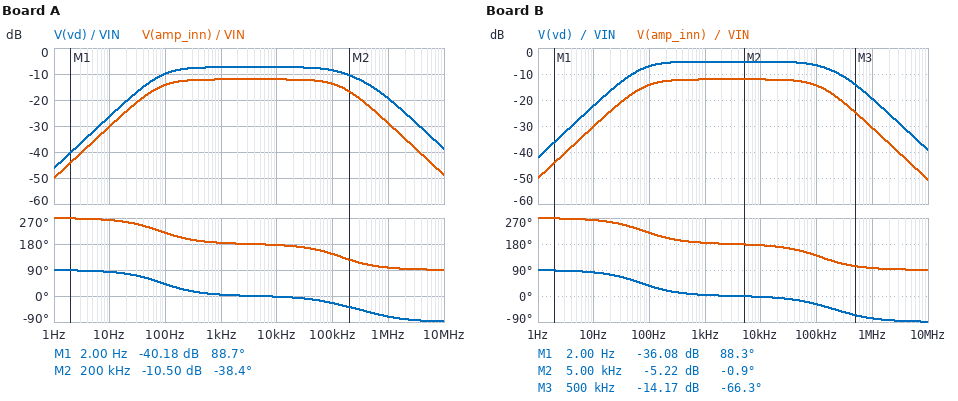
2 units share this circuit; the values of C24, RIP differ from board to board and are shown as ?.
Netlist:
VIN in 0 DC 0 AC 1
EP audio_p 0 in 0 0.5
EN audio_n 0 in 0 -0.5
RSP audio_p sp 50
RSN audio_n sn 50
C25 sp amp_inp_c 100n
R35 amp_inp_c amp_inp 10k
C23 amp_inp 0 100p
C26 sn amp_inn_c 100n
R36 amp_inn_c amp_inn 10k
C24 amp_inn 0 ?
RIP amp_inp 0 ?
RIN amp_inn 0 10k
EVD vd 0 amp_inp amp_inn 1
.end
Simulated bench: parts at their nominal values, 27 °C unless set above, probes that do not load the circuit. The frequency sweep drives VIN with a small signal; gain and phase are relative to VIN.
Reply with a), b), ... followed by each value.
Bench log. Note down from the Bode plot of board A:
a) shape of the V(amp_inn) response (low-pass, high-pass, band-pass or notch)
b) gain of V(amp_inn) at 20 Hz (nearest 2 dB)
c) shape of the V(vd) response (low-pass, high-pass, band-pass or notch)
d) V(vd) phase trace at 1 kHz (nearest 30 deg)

a) band-pass
b) -24 dB
c) band-pass
d) 0 deg
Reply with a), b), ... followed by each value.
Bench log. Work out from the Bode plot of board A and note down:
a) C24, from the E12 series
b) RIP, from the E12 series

a) 220 pF
b) 5.6 kΩ
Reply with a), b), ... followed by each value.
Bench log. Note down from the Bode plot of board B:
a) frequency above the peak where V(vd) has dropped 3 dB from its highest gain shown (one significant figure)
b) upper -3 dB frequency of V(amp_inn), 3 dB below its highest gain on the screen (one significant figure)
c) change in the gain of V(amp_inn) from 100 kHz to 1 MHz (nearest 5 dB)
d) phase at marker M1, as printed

a) 200 kHz
b) 100 kHz
c) -15 dB
d) 88.3 deg
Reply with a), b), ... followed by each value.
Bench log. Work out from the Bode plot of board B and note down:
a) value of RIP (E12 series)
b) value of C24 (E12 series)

a) 15 kΩ
b) 270 pF
